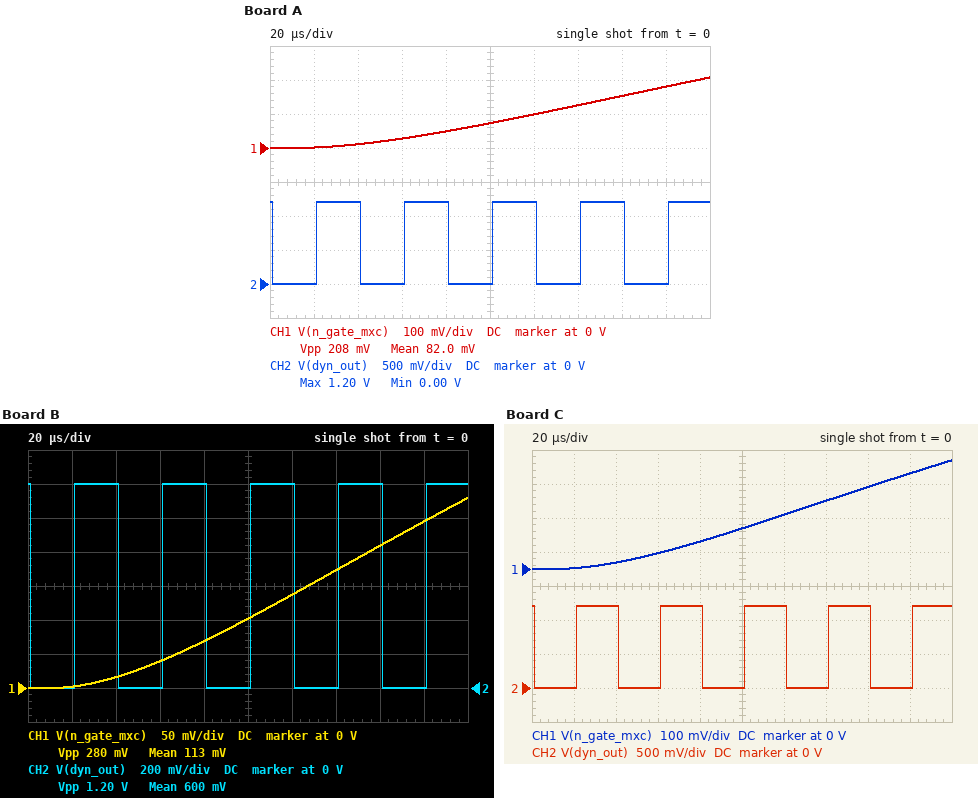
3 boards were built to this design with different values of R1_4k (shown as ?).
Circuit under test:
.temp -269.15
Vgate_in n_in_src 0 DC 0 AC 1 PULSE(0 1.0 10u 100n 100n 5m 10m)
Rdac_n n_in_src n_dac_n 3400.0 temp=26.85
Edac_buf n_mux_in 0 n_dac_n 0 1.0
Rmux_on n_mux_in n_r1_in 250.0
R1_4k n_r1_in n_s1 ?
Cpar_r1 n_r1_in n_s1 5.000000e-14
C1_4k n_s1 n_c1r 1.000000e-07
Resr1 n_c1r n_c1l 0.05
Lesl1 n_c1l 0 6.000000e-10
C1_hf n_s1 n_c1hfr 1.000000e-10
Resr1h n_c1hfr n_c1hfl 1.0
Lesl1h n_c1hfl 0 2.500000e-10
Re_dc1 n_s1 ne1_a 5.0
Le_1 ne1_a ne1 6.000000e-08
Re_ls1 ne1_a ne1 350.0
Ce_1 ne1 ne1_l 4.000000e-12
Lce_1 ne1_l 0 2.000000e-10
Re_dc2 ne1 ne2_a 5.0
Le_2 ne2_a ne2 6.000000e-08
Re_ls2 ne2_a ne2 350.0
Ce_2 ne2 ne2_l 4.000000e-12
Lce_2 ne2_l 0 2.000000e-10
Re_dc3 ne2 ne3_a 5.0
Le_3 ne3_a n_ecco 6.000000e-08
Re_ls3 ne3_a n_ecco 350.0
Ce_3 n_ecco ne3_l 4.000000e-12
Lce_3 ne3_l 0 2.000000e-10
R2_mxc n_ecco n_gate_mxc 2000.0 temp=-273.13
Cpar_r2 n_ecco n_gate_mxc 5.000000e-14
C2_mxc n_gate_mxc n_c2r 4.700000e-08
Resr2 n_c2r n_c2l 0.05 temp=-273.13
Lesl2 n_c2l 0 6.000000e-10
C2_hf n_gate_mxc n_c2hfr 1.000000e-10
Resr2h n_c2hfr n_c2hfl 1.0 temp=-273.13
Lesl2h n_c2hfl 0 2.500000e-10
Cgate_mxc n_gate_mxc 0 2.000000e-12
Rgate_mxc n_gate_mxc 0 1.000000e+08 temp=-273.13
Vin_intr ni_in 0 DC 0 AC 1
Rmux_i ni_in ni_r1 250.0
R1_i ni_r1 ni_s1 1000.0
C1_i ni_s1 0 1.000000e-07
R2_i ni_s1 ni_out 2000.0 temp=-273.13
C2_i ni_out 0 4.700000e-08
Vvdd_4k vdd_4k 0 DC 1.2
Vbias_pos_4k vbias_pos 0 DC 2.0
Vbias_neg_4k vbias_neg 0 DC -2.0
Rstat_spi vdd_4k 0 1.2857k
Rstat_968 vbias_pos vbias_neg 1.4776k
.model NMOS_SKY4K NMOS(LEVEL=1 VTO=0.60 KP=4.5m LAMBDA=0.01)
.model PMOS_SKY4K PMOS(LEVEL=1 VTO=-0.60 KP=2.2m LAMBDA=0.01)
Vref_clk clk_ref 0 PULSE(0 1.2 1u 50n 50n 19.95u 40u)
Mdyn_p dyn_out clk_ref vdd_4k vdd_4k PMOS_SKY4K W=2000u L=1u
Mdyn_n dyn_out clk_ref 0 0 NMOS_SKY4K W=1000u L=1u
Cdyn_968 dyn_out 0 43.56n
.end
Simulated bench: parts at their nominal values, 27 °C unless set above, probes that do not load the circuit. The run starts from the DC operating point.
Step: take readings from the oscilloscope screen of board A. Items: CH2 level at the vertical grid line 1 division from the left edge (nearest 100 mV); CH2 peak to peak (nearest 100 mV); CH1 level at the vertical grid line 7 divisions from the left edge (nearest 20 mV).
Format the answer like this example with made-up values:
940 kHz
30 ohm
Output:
0 V
1.2 V
120 mV
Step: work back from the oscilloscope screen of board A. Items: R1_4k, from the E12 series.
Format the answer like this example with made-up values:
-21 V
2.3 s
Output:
3.3 kΩ
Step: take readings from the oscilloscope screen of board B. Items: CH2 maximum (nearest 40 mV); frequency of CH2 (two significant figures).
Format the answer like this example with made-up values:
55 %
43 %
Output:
1.20 V
25 kHz
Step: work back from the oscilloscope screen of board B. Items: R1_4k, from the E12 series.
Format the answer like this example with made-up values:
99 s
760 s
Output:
2.2 kΩ
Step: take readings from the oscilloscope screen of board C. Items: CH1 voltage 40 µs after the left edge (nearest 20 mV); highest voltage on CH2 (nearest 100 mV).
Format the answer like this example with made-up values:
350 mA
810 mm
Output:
20 mV
1.2 V
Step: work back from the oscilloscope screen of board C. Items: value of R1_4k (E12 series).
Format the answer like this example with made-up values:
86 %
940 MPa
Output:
1.8 kΩ
